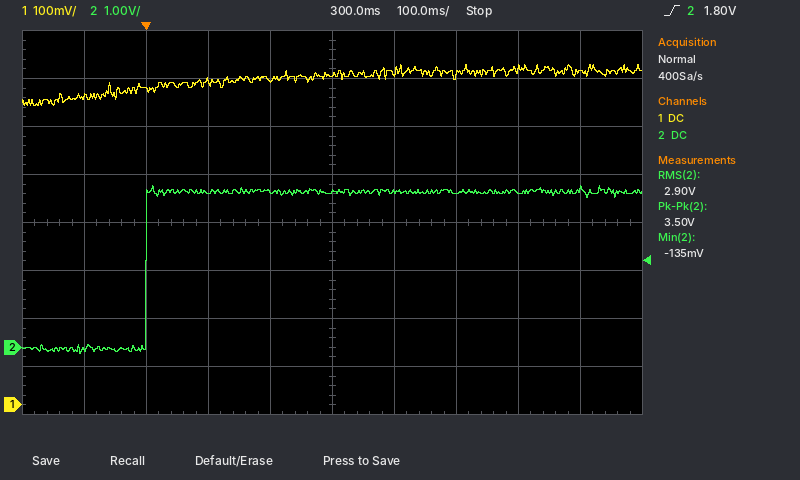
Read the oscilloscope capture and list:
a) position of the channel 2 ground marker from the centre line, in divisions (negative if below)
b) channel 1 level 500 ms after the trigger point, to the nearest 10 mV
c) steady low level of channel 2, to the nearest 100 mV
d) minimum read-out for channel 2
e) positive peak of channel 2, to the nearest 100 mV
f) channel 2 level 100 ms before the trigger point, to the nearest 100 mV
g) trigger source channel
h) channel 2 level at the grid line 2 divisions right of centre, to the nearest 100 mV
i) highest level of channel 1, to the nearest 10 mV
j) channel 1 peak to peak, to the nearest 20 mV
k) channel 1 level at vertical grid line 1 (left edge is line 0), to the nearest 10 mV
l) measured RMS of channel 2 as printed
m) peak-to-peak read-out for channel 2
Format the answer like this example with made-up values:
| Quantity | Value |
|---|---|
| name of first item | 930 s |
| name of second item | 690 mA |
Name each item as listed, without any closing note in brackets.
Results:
| Quantity | Value |
|---|---|
| position of the channel 2 ground marker from the centre line, in divisions | -2.6 div |
| channel 1 level 500 ms after the trigger point, to the nearest 10 mV | 690 mV |
| steady low level of channel 2, to the nearest 100 mV | 0.0 V |
| minimum read-out for channel 2 | -135 mV |
| positive peak of channel 2, to the nearest 100 mV | 3.4 V |
| channel 2 level 100 ms before the trigger point, to the nearest 100 mV | 0.0 V |
| trigger source channel | channel 2 |
| channel 2 level at the grid line 2 divisions right of centre, to the nearest 100 mV | 3.2 V |
| highest level of channel 1, to the nearest 10 mV | 710 mV |
| channel 1 peak to peak, to the nearest 20 mV | 80 mV |
| channel 1 level at vertical grid line 1 (left edge is line 0), to the nearest 10 mV | 640 mV |
| measured RMS of channel 2 as printed | 2.90 V |
| peak-to-peak read-out for channel 2 | 3.50 V |
